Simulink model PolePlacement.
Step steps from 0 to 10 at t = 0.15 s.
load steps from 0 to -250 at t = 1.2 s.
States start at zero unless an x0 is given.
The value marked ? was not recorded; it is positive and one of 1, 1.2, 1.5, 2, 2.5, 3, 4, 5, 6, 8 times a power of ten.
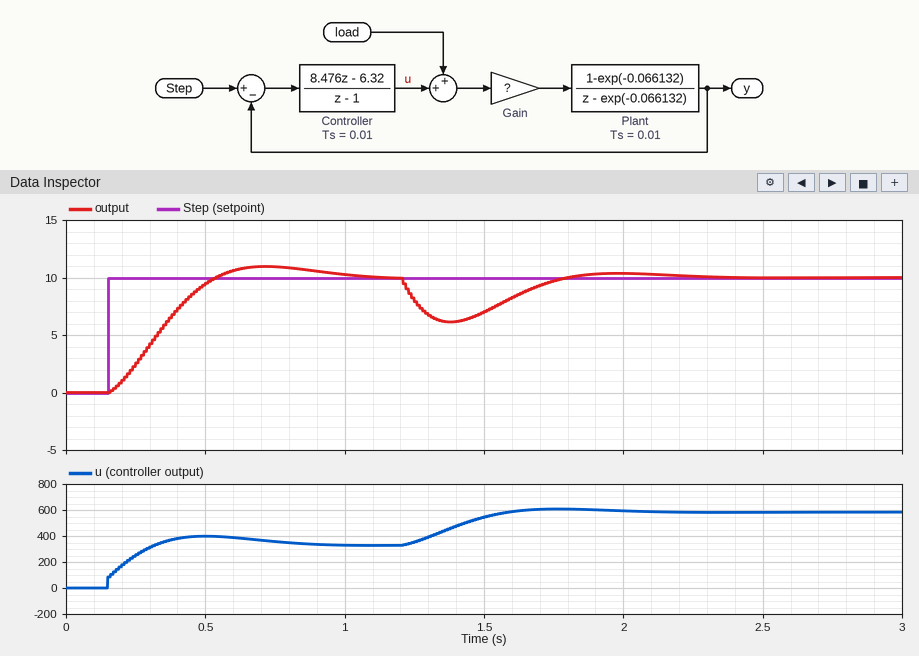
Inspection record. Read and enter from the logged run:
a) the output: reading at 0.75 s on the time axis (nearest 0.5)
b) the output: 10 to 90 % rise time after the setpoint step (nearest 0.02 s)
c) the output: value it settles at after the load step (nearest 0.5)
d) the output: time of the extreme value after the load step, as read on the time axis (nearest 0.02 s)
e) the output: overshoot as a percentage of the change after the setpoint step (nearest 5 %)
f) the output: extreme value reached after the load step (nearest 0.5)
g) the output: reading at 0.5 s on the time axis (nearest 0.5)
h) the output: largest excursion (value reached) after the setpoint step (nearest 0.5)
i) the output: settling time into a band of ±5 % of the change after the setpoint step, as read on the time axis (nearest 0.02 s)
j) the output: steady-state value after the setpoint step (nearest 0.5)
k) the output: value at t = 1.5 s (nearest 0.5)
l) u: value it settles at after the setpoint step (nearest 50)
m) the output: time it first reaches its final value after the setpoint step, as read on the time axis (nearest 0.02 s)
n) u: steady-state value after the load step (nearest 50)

11.0
0.28 s
10.0
1.38 s
10 %
6.0
9.5
11.0
0.92 s
10.0
7.0
350
0.54 s
600
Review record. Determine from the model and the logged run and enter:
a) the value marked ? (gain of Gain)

0.03
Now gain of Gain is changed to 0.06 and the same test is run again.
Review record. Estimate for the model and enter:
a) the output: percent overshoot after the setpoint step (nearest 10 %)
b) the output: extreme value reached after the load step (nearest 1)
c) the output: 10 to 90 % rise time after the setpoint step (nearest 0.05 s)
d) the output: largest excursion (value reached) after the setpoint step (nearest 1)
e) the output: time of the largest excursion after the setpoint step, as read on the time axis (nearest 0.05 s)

20 %
4
0.15 s
12
0.50 s
